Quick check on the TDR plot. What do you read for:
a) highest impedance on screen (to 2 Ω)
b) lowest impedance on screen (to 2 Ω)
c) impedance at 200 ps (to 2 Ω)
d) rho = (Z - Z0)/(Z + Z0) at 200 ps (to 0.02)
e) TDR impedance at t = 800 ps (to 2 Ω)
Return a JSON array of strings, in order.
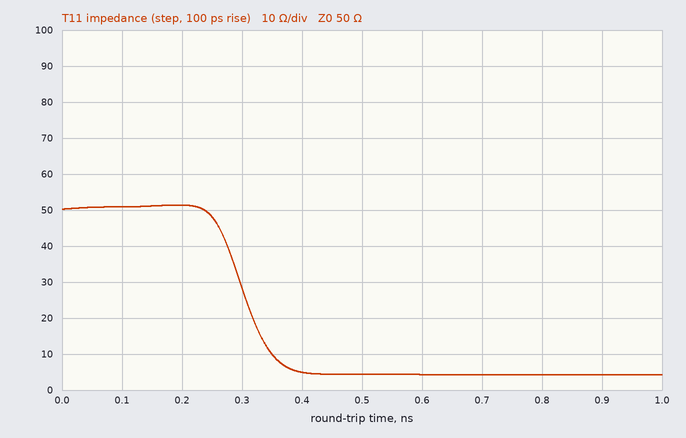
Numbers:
["52 Ω", "4 Ω", "52 Ω", "+0.02", "4 Ω"]
